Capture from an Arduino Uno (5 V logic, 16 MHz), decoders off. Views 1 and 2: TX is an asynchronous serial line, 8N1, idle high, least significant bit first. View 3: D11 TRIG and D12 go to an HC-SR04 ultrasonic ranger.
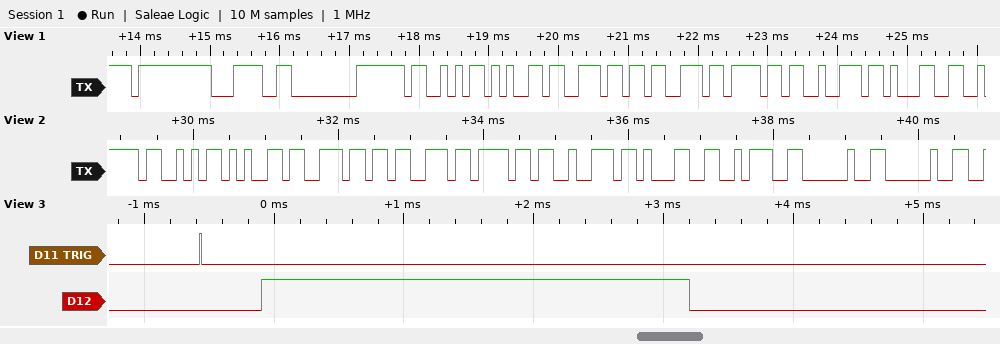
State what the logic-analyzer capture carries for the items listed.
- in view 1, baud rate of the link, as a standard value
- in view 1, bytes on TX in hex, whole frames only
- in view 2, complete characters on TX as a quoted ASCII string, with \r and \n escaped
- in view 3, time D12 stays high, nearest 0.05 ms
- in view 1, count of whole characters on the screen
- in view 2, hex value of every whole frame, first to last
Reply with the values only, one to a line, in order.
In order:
9600 baud
0xFF 0x3C 0x00 0x53 0x65 0x6E 0x73 0x6F 0x72 0x31
"Sensor1:  "
3.30 ms
10
53 65 6E 73 6F 72 31 3A 20 20
